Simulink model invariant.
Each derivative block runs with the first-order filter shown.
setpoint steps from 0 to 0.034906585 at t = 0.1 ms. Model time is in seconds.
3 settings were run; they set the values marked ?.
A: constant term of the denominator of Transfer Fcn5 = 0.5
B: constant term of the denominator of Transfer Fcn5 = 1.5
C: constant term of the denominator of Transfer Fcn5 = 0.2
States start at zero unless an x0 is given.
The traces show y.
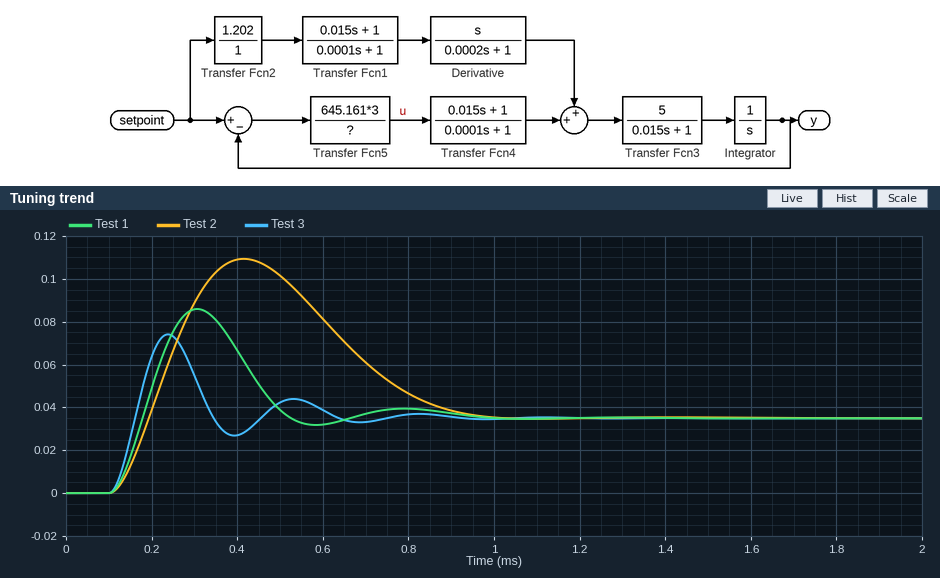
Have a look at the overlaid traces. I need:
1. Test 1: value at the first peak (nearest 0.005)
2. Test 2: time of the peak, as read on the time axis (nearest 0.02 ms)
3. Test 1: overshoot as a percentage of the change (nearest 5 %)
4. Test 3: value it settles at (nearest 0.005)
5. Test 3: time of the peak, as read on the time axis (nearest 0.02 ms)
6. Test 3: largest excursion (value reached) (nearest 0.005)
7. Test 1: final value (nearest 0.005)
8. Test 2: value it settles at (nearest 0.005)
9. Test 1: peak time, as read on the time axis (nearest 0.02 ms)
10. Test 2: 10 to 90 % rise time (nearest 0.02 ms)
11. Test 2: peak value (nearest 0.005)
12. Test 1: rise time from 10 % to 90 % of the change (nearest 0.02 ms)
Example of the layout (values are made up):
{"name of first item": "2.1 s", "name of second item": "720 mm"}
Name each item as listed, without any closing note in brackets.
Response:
{"Test 1: value at the first peak": "0.085", "Test 2: time of the peak, as read on the time axis": "0.42 ms", "Test 1: overshoot as a percentage of the change": "145 %", "Test 3: value it settles at": "0.035", "Test 3: time of the peak, as read on the time axis": "0.24 ms", "Test 3: largest excursion (value reached)": "0.075", "Test 1: final value": "0.035", "Test 2: value it settles at": "0.035", "Test 1: peak time, as read on the time axis": "0.30 ms", "Test 2: 10 to 90 % rise time": "0.06 ms", "Test 2: peak value": "0.110", "Test 1: rise time from 10 % to 90 % of the change": "0.06 ms"}
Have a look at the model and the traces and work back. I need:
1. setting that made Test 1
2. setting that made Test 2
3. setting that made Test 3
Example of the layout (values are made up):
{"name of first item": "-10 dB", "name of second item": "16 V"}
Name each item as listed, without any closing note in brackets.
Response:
{"setting that made Test 1": "A", "setting that made Test 2": "B", "setting that made Test 3": "C"}
